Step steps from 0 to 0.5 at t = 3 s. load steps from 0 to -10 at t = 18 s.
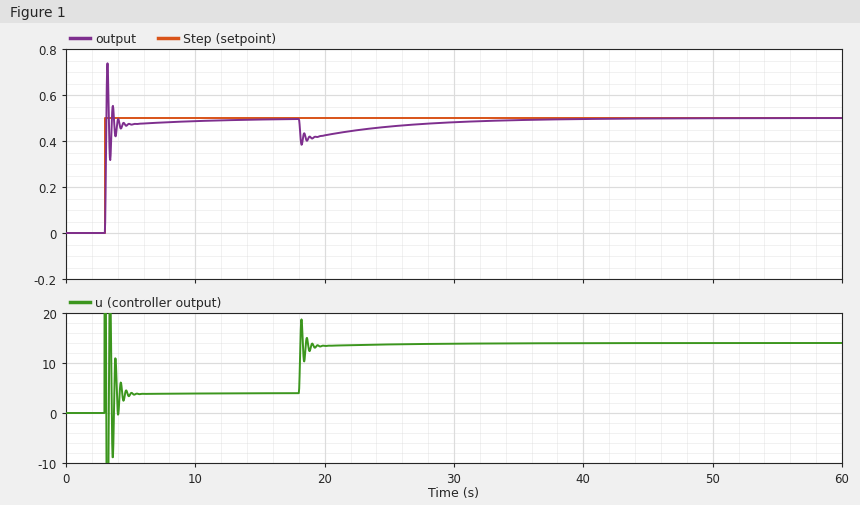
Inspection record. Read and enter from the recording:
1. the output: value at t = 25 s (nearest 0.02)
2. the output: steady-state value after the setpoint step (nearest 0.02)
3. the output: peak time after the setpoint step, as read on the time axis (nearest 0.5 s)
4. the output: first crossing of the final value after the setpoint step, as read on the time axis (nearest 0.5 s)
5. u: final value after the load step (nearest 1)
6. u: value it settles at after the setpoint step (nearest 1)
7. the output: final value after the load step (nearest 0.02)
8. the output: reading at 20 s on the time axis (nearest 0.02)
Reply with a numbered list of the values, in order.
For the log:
1. 0.46
2. 0.50
3. 3.0 s
4. 3.0 s
5. 14
6. 4
7. 0.50
8. 0.42
